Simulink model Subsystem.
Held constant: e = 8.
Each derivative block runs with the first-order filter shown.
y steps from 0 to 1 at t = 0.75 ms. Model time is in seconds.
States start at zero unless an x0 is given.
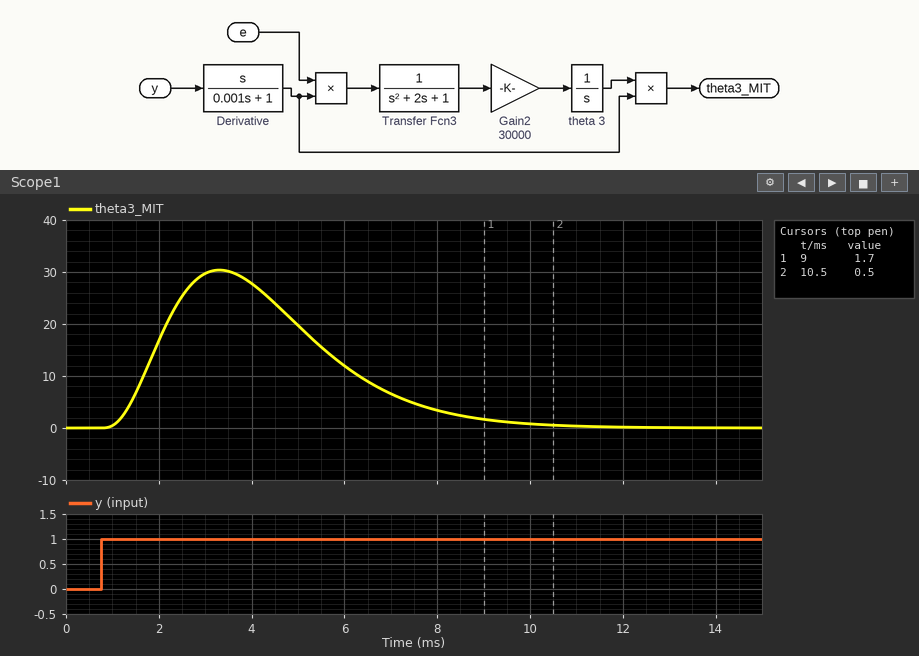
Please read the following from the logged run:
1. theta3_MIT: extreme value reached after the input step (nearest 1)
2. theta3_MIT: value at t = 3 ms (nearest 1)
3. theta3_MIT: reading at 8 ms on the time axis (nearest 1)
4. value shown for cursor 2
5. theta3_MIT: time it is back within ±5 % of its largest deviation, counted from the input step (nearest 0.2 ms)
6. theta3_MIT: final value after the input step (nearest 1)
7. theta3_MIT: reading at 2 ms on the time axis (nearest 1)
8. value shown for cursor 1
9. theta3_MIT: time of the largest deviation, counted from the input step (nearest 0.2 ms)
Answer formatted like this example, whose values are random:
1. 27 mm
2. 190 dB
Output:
1. 30
2. 30
3. 3
4. 0.5
5. 8.4 ms
6. 0
7. 17
8. 1.7
9. 2.6 ms
